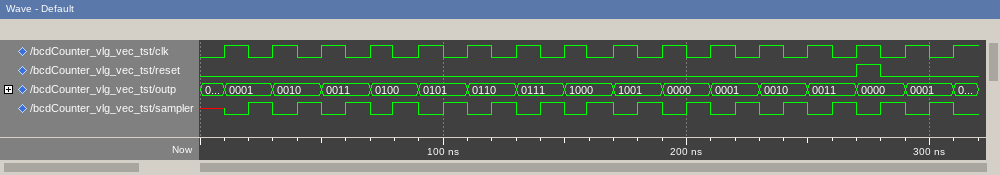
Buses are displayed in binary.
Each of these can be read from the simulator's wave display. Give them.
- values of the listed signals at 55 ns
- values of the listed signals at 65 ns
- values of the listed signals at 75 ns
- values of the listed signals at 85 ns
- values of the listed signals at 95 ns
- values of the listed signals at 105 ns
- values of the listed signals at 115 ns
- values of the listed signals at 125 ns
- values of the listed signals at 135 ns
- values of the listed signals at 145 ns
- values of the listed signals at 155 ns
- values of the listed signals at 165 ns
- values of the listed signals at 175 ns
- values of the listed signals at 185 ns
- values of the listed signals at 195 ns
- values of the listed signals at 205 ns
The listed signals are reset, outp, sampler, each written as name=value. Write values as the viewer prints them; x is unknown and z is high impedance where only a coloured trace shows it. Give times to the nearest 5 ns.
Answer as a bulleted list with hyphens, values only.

- reset=0, outp=0011, sampler=0
- reset=0, outp=0011, sampler=1
- reset=0, outp=0100, sampler=0
- reset=0, outp=0100, sampler=1
- reset=0, outp=0101, sampler=0
- reset=0, outp=0101, sampler=1
- reset=0, outp=0110, sampler=0
- reset=0, outp=0110, sampler=1
- reset=0, outp=0111, sampler=0
- reset=0, outp=0111, sampler=1
- reset=0, outp=1000, sampler=0
- reset=0, outp=1000, sampler=1
- reset=0, outp=1001, sampler=0
- reset=0, outp=1001, sampler=1
- reset=0, outp=0000, sampler=0
- reset=0, outp=0000, sampler=1
